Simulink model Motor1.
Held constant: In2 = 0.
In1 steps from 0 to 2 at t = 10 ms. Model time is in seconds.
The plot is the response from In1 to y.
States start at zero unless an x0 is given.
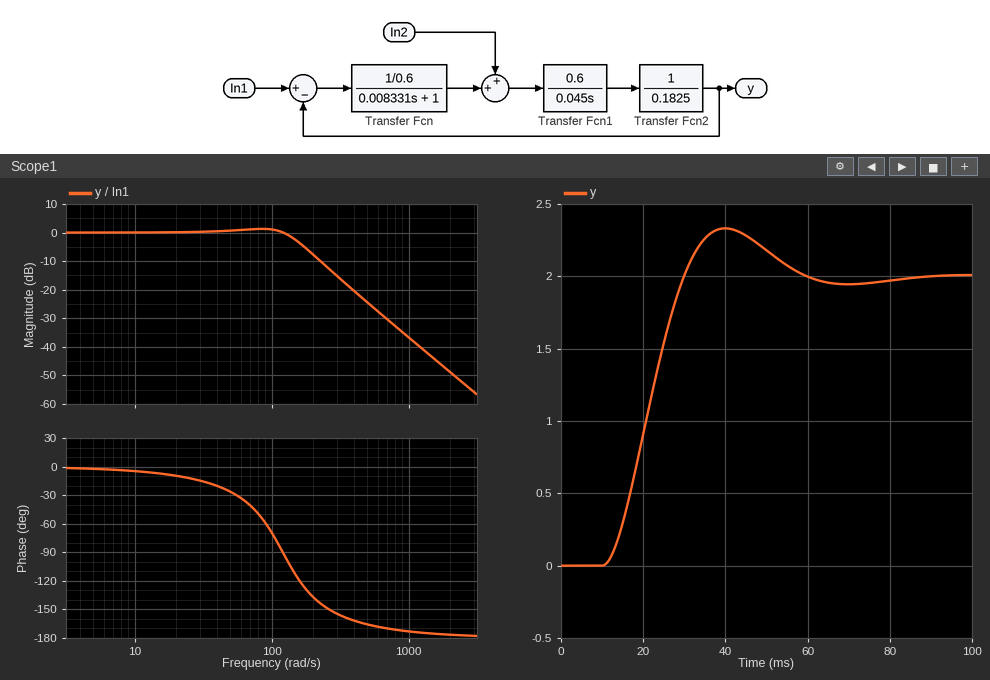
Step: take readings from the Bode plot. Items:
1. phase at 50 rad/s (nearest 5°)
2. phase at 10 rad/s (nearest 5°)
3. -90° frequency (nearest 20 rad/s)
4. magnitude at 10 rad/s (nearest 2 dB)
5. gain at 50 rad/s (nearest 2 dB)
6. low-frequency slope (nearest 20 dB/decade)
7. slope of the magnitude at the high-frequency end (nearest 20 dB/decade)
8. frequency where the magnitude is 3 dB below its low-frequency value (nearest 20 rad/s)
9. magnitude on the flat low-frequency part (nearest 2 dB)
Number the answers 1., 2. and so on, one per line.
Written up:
1. -25°
2. -5°
3. 120 rad/s
4. 0 dB
5. 0 dB
6. 0 dB/decade
7. -40 dB/decade
8. 160 rad/s
9. 0 dB
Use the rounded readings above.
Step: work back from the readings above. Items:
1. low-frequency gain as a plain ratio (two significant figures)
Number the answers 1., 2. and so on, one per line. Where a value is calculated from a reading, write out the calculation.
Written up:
1. 10^(0 / 20) = 1.0
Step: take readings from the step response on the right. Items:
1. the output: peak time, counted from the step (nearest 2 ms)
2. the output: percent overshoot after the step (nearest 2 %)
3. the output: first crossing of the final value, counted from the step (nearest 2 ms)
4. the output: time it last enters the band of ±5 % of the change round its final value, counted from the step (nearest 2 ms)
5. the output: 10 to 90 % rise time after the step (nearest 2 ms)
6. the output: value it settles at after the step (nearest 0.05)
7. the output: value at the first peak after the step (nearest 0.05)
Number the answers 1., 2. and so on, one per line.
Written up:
1. 30 ms
2. 16 %
3. 20 ms
4. 44 ms
5. 14 ms
6. 2.00
7. 2.35
